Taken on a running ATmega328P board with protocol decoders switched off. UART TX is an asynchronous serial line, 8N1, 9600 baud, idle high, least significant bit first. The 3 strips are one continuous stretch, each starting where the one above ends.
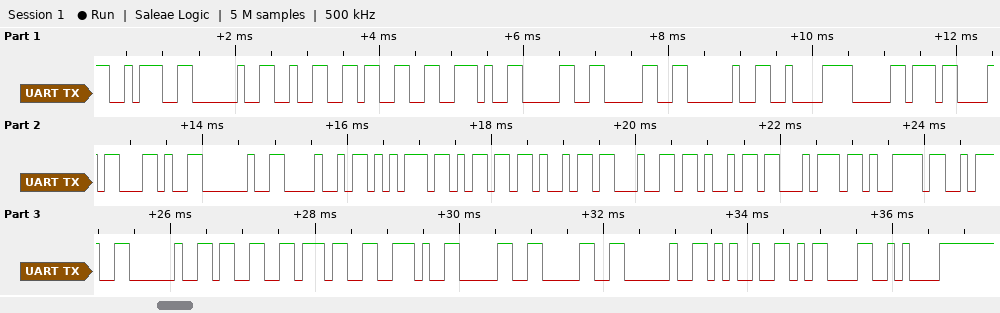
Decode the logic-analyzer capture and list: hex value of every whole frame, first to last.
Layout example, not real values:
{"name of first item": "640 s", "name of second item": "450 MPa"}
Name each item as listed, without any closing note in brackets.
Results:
{"hex value of every whole frame, first to last": "0x3A 0x20 0x32 0x33 0x2E 0x30 0x30 0x20 0xC2 0xB0 0x43 0x2C 0x20 0x48 0x75 0x6D 0x69 0x64 0x69 0x74 0x79 0x3A 0x20 0x33 0x37 0x2E 0x30 0x30 0x20 0x25 0x0D 0x0A"}
